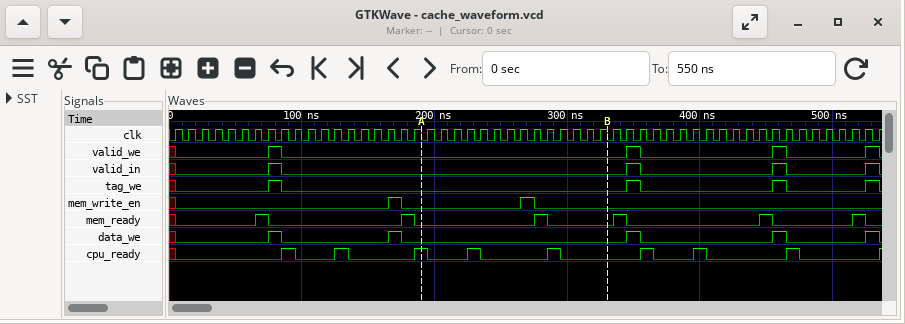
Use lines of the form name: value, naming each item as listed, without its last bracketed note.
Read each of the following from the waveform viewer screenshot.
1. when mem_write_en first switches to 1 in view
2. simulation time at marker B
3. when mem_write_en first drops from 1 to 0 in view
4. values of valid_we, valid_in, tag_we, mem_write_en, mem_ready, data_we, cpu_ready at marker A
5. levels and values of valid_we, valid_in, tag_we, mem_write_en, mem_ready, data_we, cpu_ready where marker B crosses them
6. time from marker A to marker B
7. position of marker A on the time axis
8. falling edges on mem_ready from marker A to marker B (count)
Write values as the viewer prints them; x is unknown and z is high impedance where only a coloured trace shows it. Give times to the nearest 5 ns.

when mem_write_en first switches to 1 in view: 165 ns
simulation time at marker B: 330 ns
when mem_write_en first drops from 1 to 0 in view: 175 ns
values of valid_we, valid_in, tag_we, mem_write_en, mem_ready, data_we, cpu_ready at marker A: valid_we=0, valid_in=0, tag_we=0, mem_write_en=0, mem_ready=0, data_we=0, cpu_ready=1
levels and values of valid_we, valid_in, tag_we, mem_write_en, mem_ready, data_we, cpu_ready where marker B crosses them: valid_we=0, valid_in=0, tag_we=0, mem_write_en=0, mem_ready=0, data_we=0, cpu_ready=0
time from marker A to marker B: 140 ns
position of marker A on the time axis: 190 ns
falling edges on mem_ready from marker A to marker B: 1
